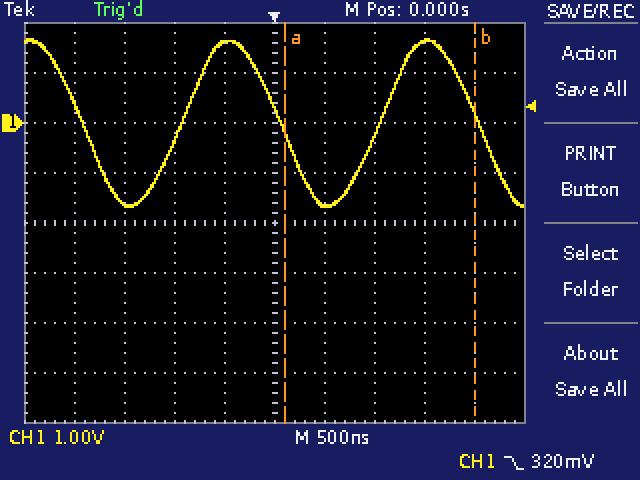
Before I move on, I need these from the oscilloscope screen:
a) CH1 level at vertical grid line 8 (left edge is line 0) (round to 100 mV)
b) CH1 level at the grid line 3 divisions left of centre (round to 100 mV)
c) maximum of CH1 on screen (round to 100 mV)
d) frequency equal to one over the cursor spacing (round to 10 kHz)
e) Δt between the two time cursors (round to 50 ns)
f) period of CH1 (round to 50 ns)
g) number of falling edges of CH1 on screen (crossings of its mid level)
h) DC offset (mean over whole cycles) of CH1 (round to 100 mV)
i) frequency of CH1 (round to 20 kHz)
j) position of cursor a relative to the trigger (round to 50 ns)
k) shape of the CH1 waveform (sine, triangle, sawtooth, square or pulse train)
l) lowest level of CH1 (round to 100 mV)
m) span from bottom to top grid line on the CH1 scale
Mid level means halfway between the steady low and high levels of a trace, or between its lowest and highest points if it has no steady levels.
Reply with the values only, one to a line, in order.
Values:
1.6 V
-1.6 V
1.7 V
530 kHz
1.90 µs
2.00 µs
3
0.0 V
500 kHz
+100 ns
sine
-1.7 V
8 V
